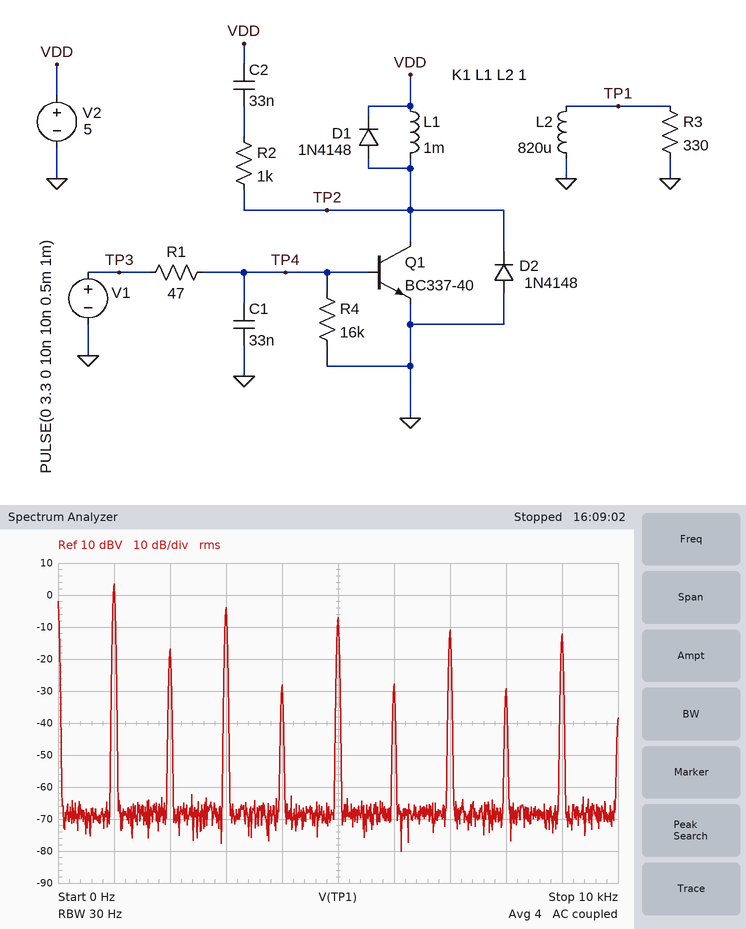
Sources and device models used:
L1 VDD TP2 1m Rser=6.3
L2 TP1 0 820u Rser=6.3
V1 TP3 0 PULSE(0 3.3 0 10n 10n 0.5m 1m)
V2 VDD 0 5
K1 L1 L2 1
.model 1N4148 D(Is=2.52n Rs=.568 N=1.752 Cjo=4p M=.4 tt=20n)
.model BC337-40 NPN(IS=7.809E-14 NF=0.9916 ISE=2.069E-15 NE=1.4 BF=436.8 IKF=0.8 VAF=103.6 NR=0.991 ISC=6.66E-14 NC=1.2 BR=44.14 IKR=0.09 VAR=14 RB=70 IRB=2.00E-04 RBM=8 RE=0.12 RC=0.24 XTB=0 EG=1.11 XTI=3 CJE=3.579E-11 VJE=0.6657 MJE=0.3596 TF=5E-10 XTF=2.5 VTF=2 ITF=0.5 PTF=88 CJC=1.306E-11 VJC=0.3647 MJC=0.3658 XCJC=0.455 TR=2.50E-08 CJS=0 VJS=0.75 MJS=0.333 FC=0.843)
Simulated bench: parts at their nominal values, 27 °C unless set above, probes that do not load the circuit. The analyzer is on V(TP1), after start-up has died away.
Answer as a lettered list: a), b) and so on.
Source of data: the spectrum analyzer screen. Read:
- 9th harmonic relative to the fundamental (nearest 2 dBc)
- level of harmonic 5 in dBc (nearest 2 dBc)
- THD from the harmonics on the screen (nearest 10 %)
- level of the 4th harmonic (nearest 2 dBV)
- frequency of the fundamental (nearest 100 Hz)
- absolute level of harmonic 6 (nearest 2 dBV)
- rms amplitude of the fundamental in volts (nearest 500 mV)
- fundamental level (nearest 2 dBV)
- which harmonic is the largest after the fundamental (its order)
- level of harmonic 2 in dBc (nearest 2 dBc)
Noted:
a) -16 dBc
b) -10 dBc
c) 60 %
d) -28 dBV
e) 1.0 kHz
f) -28 dBV
g) 1.5 V
h) 4 dBV
i) 3
j) -20 dBc
